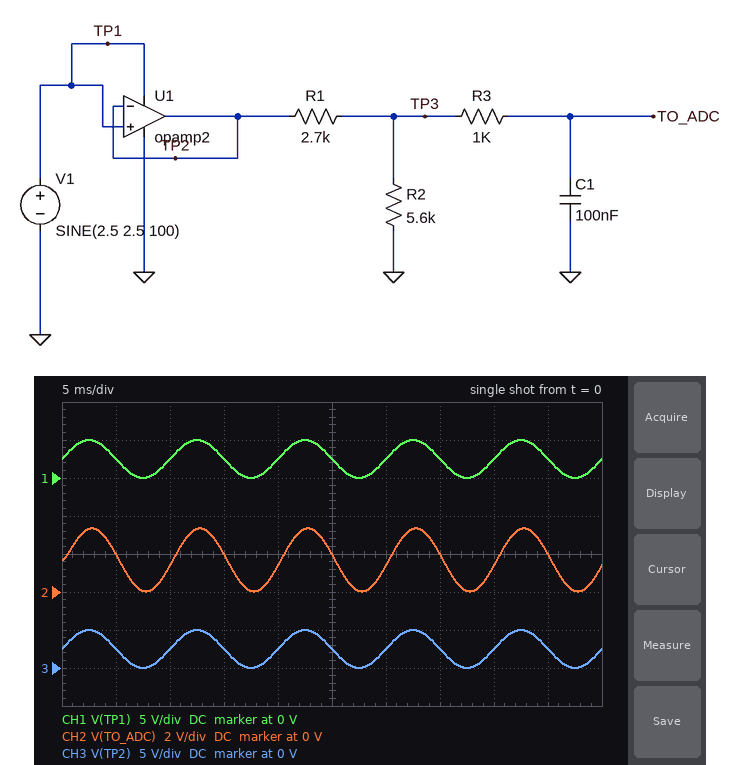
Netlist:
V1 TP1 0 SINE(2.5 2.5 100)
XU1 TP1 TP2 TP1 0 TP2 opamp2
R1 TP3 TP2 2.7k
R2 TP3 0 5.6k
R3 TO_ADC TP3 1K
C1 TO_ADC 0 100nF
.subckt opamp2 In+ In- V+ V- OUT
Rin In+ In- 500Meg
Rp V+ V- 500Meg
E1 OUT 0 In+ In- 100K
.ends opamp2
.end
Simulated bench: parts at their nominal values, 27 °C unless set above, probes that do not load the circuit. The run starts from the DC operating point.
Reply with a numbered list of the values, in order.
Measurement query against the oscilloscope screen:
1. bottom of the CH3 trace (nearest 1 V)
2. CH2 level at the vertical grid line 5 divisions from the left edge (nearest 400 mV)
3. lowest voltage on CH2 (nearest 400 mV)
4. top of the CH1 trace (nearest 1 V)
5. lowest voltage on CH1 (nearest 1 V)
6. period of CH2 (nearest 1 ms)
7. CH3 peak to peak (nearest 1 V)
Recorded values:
1. 0 V
2. 2.0 V
3. 0 V
4. 5 V
5. 0 V
6. 10 ms
7. 5 V
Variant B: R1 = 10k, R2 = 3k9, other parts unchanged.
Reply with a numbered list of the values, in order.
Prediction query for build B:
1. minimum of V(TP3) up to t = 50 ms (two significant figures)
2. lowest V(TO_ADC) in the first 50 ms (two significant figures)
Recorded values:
1. 18 mV
2. 19 mV
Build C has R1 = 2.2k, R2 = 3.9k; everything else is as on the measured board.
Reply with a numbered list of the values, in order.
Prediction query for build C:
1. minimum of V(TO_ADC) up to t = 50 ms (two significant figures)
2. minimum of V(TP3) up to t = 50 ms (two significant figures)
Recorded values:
1. 18 mV
2. 15 mV
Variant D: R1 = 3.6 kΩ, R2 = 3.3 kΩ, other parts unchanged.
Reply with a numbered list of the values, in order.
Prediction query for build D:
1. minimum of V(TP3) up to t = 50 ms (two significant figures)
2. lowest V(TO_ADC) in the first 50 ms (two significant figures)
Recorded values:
1. 15 mV
2. 17 mV
